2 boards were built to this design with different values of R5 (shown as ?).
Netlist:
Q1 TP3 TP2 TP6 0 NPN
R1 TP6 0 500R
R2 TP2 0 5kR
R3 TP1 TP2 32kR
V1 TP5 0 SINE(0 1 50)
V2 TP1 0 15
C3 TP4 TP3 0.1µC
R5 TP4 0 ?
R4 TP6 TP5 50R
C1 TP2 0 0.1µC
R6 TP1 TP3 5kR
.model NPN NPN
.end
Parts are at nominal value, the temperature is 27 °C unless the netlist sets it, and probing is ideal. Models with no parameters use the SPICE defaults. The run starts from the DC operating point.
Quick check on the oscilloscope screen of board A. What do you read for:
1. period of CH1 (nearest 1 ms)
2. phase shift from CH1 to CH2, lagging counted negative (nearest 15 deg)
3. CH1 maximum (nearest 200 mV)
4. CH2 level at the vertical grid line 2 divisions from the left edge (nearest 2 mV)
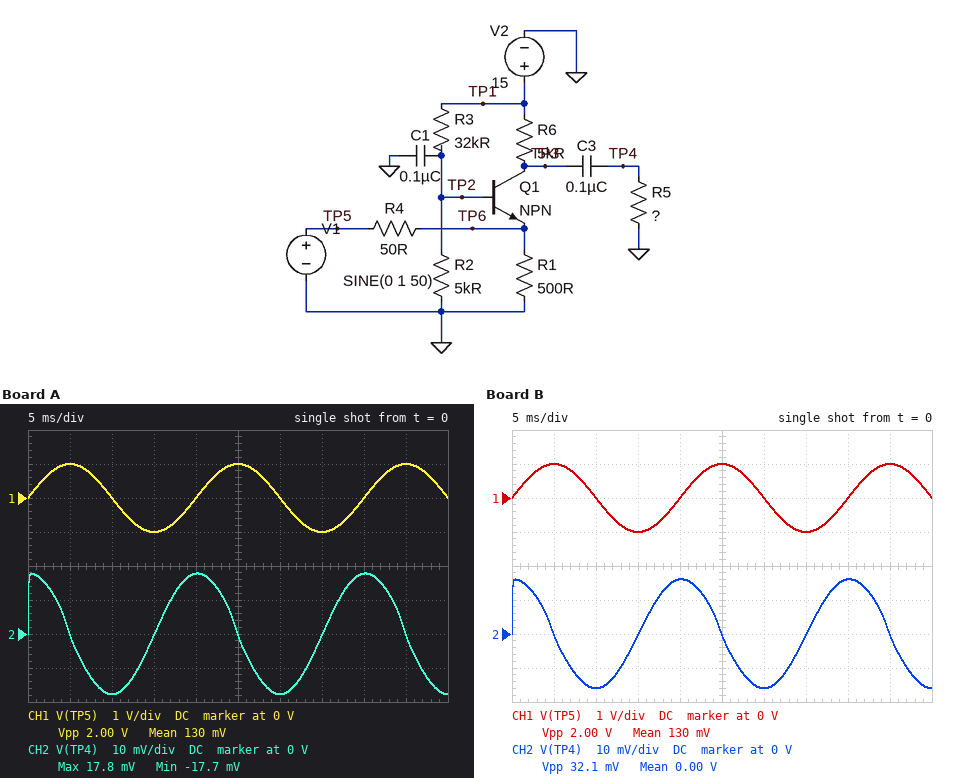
20 ms
90 deg
1.0 V
-18 mV
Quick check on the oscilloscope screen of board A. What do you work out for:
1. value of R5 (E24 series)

620 Ω
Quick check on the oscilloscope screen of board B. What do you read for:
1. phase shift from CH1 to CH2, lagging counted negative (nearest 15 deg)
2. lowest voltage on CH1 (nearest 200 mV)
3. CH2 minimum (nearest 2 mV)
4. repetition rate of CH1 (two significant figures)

90 deg
-1.0 V
-16 mV
50 Hz
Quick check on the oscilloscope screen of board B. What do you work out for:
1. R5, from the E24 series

560 Ω
